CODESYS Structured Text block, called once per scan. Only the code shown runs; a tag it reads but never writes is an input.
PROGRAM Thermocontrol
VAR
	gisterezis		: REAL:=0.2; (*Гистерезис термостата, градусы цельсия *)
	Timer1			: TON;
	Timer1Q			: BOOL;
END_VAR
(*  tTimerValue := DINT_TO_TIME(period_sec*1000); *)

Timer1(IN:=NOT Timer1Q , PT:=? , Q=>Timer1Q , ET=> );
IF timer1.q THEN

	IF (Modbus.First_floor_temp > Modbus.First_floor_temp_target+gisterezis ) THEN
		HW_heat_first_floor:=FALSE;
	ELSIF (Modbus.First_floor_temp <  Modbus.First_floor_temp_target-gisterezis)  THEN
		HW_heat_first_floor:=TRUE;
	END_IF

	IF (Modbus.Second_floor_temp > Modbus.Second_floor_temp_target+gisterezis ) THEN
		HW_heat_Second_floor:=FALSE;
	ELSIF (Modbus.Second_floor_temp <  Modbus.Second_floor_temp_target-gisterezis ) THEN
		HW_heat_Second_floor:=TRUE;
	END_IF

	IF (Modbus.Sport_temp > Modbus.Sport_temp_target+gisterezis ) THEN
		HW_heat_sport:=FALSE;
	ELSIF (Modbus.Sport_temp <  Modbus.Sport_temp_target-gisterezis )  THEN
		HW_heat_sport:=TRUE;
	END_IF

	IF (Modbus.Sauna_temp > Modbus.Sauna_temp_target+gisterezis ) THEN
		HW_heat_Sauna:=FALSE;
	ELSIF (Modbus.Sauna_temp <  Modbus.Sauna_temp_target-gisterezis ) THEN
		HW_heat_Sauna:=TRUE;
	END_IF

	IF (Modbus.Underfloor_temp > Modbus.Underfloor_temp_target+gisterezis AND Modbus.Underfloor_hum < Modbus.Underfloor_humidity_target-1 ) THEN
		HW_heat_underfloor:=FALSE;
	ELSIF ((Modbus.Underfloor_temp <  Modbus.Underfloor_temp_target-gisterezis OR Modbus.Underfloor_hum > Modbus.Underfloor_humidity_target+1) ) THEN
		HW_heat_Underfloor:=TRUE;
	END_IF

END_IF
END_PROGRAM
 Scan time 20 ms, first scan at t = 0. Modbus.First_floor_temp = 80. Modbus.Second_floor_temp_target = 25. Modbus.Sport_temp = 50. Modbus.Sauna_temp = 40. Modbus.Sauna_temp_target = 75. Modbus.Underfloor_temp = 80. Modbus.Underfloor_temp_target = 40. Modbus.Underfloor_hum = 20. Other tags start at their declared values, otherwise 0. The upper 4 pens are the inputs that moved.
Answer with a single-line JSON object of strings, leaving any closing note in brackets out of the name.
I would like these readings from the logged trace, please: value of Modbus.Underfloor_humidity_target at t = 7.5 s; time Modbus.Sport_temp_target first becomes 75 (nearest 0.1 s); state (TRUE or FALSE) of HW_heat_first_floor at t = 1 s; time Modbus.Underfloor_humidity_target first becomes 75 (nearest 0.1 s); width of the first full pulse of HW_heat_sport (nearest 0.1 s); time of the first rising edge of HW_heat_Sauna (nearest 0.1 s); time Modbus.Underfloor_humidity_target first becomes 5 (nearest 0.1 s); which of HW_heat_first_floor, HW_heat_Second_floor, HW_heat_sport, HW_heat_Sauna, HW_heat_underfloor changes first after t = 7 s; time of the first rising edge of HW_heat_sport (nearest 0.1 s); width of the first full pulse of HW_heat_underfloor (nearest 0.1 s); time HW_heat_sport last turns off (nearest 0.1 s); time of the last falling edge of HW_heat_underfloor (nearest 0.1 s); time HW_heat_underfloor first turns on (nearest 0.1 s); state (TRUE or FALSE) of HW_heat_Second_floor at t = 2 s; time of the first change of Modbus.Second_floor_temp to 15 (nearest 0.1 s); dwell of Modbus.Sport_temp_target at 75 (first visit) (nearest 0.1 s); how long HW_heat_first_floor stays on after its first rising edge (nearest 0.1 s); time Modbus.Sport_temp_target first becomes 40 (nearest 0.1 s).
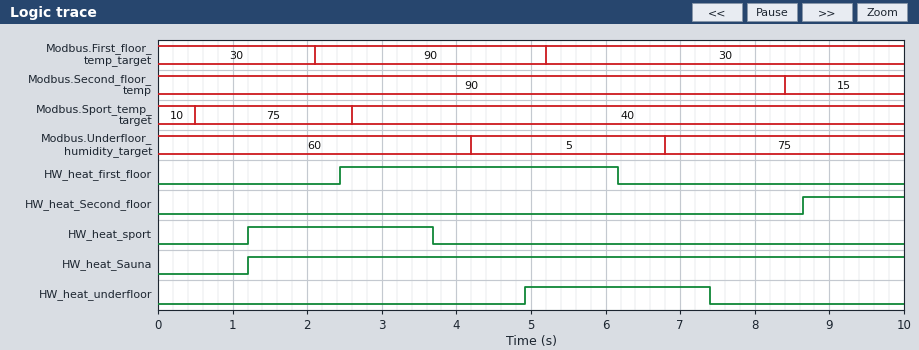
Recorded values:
{"value of Modbus.Underfloor_humidity_target at t = 7.5 s": "75", "time Modbus.Sport_temp_target first becomes 75": "0.5 s", "state (TRUE or FALSE) of HW_heat_first_floor at t = 1 s": "FALSE", "time Modbus.Underfloor_humidity_target first becomes 75": "6.8 s", "width of the first full pulse of HW_heat_sport": "2.5 s", "time of the first rising edge of HW_heat_Sauna": "1.2 s", "time Modbus.Underfloor_humidity_target first becomes 5": "4.2 s", "which of HW_heat_first_floor, HW_heat_Second_floor, HW_heat_sport, HW_heat_Sauna, HW_heat_underfloor changes first after t = 7 s": "HW_heat_underfloor", "time of the first rising edge of HW_heat_sport": "1.2 s", "width of the first full pulse of HW_heat_underfloor": "2.5 s", "time HW_heat_sport last turns off": "3.7 s", "time of the last falling edge of HW_heat_underfloor": "7.4 s", "time HW_heat_underfloor first turns on": "4.9 s", "state (TRUE or FALSE) of HW_heat_Second_floor at t = 2 s": "FALSE", "time of the first change of Modbus.Second_floor_temp to 15": "8.4 s", "dwell of Modbus.Sport_temp_target at 75 (first visit)": "2.1 s", "how long HW_heat_first_floor stays on after its first rising edge": "3.7 s", "time Modbus.Sport_temp_target first becomes 40": "2.6 s"}
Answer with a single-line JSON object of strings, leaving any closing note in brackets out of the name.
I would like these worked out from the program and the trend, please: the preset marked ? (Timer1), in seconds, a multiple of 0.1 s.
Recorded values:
{"the preset marked ? (Timer1), in seconds, a multiple of 0.1 s": "1.2 s"}
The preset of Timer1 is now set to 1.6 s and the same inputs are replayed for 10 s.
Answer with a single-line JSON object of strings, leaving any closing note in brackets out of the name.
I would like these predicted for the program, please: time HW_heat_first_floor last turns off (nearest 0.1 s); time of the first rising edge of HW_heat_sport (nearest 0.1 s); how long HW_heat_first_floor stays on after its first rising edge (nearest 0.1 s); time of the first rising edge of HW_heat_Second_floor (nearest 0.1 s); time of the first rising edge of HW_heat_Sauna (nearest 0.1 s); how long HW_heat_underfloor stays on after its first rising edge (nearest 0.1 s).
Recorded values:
{"time HW_heat_first_floor last turns off": "6.5 s", "time of the first rising edge of HW_heat_sport": "1.6 s", "how long HW_heat_first_floor stays on after its first rising edge": "3.3 s", "time of the first rising edge of HW_heat_Second_floor": "9.8 s", "time of the first rising edge of HW_heat_Sauna": "1.6 s", "how long HW_heat_underfloor stays on after its first rising edge": "3.3 s"}
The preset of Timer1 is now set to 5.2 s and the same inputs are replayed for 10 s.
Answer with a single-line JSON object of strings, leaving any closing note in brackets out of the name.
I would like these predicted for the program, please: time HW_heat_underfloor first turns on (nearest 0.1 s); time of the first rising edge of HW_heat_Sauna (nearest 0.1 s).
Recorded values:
{"time HW_heat_underfloor first turns on": "5.2 s", "time of the first rising edge of HW_heat_Sauna": "5.2 s"}
